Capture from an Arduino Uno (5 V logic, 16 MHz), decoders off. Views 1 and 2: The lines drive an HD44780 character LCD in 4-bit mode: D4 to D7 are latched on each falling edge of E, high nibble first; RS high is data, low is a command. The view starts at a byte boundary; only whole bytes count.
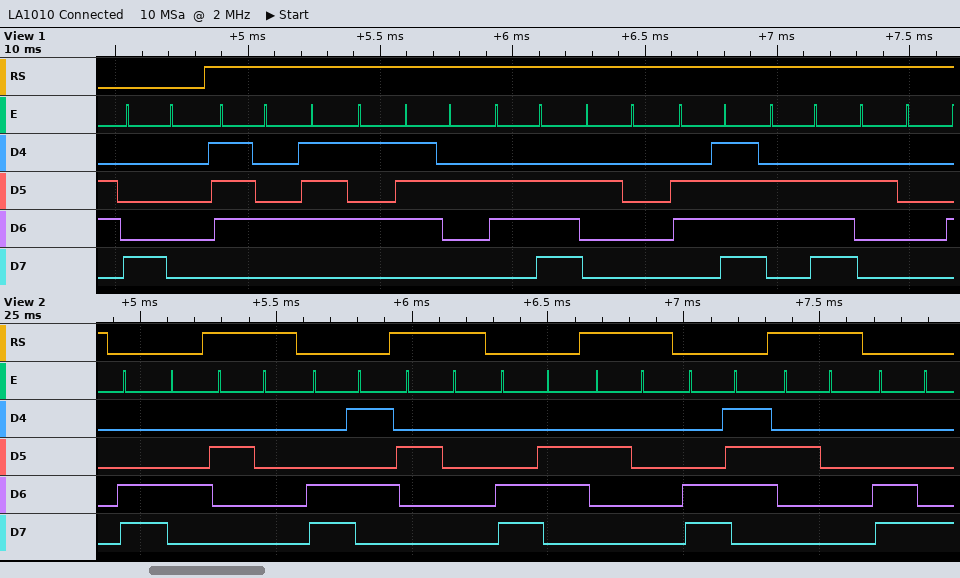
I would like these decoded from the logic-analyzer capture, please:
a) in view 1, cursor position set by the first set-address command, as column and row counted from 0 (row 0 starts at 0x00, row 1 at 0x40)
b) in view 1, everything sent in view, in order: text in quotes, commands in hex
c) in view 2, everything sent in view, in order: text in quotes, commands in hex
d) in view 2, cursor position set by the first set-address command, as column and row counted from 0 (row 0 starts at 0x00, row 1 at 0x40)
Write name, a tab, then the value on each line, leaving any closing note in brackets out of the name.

in view 1, cursor position set by the first set-address command, as column and row counted from 0	column 0, row 0
in view 1, everything sent in view, in order: text in quotes, commands in hex	0x80 "turn on "
in view 2, everything sent in view, in order: text in quotes, commands in hex	0xC4 " " 0xC5 " " 0xC6 " " 0xC7 " " 0xC8
in view 2, cursor position set by the first set-address command, as column and row counted from 0	column 4, row 1
